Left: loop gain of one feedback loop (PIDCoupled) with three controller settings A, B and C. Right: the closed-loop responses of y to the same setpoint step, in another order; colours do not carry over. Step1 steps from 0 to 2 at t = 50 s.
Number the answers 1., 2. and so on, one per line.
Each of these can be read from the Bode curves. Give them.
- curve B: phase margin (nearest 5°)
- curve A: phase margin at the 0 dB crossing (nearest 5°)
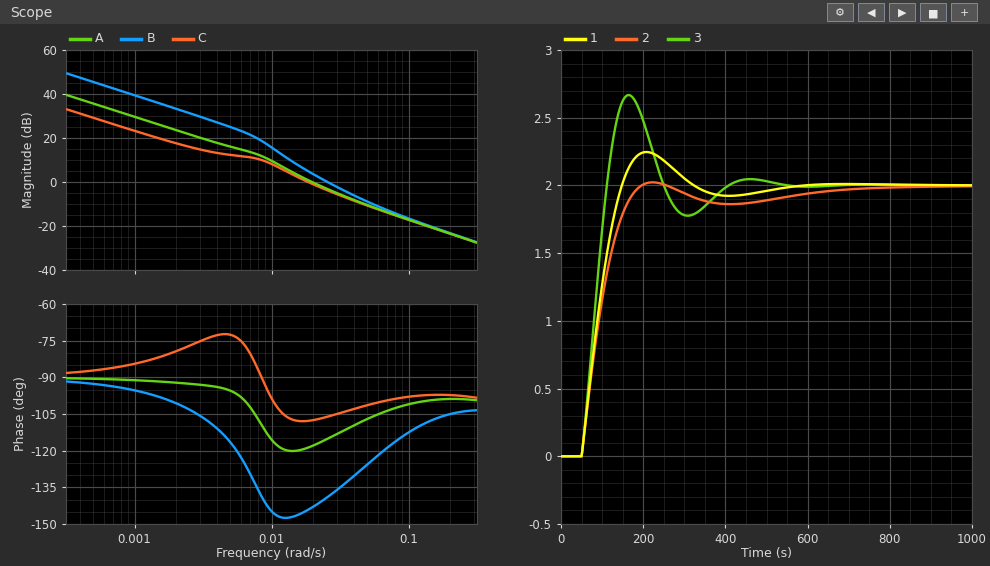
1. 40°
2. 60°
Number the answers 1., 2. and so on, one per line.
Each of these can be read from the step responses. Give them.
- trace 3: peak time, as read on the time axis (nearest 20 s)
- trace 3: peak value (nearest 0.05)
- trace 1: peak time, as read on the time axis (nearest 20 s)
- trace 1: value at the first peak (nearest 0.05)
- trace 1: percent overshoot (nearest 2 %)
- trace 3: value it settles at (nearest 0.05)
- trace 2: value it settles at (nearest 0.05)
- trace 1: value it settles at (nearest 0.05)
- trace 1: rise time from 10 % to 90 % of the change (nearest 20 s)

1. 160 s
2. 2.65
3. 200 s
4. 2.25
5. 12 %
6. 2.00
7. 2.00
8. 2.00
9. 80 s
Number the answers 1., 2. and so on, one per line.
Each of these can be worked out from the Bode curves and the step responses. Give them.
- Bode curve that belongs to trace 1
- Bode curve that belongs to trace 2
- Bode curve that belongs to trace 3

1. A
2. C
3. B
